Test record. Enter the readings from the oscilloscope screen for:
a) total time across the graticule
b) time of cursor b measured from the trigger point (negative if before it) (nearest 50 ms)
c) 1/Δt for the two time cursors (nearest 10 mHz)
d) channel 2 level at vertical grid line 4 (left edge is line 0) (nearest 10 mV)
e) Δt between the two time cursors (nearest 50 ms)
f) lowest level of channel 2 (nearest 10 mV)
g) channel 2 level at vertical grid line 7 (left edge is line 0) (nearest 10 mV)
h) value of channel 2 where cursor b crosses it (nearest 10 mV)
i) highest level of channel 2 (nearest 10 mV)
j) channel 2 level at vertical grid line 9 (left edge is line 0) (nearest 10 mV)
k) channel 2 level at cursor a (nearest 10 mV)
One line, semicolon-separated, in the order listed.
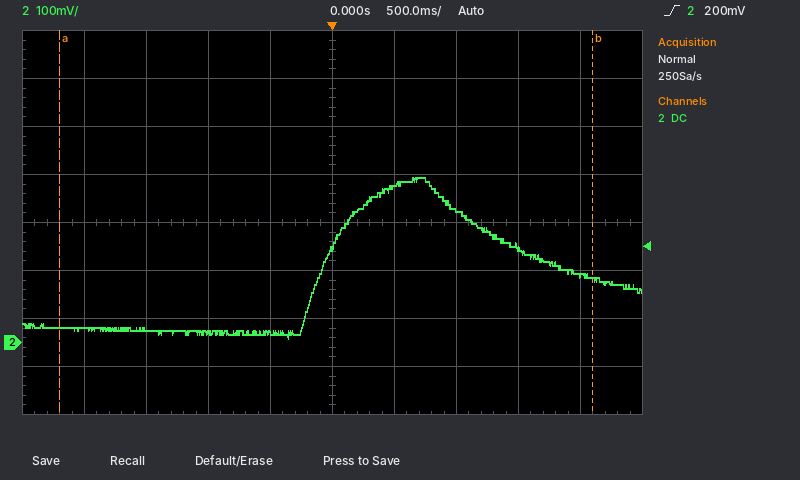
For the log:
5 s; +2.10 s; 230 mHz; 20 mV; 4.30 s; 10 mV; 280 mV; 130 mV; 340 mV; 140 mV; 30 mV
